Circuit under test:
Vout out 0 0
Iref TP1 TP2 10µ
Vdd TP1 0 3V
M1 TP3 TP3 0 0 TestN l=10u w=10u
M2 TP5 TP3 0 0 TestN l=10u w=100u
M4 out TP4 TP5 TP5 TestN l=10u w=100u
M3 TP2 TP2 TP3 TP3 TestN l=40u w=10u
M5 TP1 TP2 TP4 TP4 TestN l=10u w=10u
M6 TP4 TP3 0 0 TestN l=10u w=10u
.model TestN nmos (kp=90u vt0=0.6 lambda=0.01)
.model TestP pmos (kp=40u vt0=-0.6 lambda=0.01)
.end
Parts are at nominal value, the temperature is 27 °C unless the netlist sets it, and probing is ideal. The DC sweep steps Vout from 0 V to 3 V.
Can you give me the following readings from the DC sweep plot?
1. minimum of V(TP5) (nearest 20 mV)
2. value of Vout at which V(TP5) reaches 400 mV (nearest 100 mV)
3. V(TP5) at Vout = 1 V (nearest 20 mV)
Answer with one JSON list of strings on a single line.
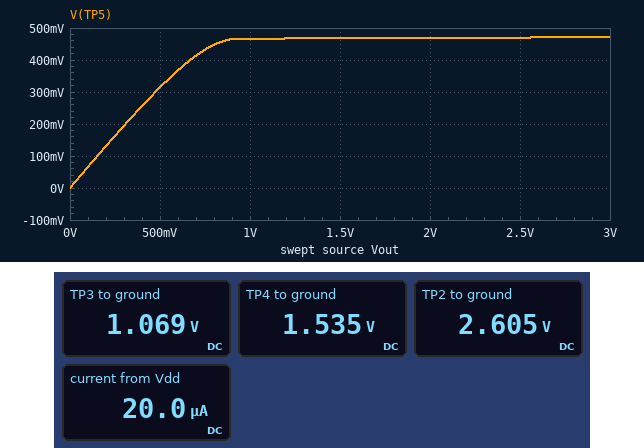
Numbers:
["0 V", "700 mV", "460 mV"]
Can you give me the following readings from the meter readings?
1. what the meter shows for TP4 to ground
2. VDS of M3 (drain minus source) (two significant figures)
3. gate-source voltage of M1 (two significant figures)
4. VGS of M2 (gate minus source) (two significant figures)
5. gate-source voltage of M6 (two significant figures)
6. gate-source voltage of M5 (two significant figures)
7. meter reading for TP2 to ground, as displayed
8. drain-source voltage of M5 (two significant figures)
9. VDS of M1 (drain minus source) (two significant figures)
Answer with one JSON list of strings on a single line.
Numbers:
["1.535 V", "1.5 V", "1.1 V", "1.1 V", "1.1 V", "1.1 V", "2.605 V", "1.5 V", "1.1 V"]
